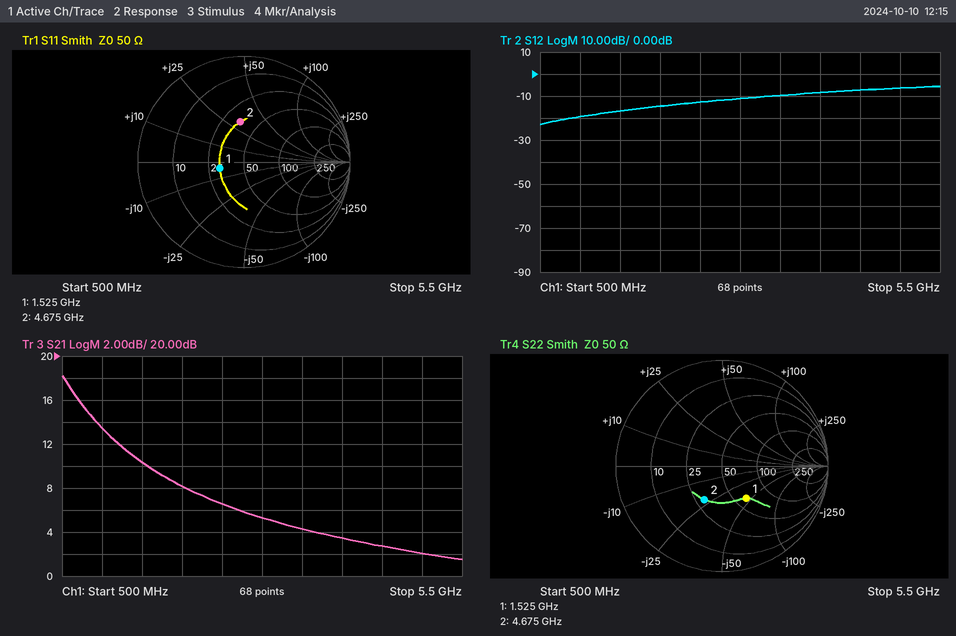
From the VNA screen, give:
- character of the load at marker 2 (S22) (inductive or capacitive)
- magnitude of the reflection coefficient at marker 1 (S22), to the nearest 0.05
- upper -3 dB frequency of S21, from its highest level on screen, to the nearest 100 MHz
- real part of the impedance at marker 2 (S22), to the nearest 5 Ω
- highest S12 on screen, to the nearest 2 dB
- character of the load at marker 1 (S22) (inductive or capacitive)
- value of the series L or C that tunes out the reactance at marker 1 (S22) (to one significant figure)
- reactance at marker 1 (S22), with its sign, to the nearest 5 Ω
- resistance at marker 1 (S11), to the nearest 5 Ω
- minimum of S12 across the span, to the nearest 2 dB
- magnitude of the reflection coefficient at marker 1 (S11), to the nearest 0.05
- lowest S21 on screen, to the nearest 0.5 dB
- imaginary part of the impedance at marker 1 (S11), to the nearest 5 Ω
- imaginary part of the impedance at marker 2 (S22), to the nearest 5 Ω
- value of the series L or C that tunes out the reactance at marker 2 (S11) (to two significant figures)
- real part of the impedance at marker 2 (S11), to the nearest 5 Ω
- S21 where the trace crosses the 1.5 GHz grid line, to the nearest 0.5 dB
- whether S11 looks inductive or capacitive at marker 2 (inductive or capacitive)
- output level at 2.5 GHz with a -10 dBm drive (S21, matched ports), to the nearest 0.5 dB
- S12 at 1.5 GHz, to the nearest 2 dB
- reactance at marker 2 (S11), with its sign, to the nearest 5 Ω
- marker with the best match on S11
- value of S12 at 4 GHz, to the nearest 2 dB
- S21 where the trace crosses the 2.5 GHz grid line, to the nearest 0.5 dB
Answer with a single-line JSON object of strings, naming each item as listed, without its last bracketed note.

{"character of the load at marker 2 (S22)": "capacitive", "magnitude of the reflection coefficient at marker 1 (S22), to the nearest 0.05": "0.40", "upper -3 dB frequency of S21, from its highest level on screen, to the nearest 100 MHz": "800 MHz", "real part of the impedance at marker 2 (S22), to the nearest 5 Ω": "30 Ω", "highest S12 on screen, to the nearest 2 dB": "-6 dB", "character of the load at marker 1 (S22)": "capacitive", "value of the series L or C that tunes out the reactance at marker 1 (S22)": "5 nH", "reactance at marker 1 (S22), with its sign, to the nearest 5 Ω": "-45 Ω", "resistance at marker 1 (S11), to the nearest 5 Ω": "30 Ω", "minimum of S12 across the span, to the nearest 2 dB": "-22 dB", "magnitude of the reflection coefficient at marker 1 (S11), to the nearest 0.05": "0.25", "lowest S21 on screen, to the nearest 0.5 dB": "1.5 dB", "imaginary part of the impedance at marker 1 (S11), to the nearest 5 Ω": "-5 Ω", "imaginary part of the impedance at marker 2 (S22), to the nearest 5 Ω": "-20 Ω", "value of the series L or C that tunes out the reactance at marker 2 (S11)": "1.1 pF", "real part of the impedance at marker 2 (S11), to the nearest 5 Ω": "35 Ω", "S21 where the trace crosses the 1.5 GHz grid line, to the nearest 0.5 dB": "10.5 dB", "whether S11 looks inductive or capacitive at marker 2": "inductive", "output level at 2.5 GHz with a -10 dBm drive (S21, matched ports), to the nearest 0.5 dB": "-3.5 dBm", "S12 at 1.5 GHz, to the nearest 2 dB": "-16 dB", "reactance at marker 2 (S11), with its sign, to the nearest 5 Ω": "+30 Ω", "marker with the best match on S11": "marker 1", "value of S12 at 4 GHz, to the nearest 2 dB": "-8 dB", "S21 where the trace crosses the 2.5 GHz grid line, to the nearest 0.5 dB": "6.5 dB"}
